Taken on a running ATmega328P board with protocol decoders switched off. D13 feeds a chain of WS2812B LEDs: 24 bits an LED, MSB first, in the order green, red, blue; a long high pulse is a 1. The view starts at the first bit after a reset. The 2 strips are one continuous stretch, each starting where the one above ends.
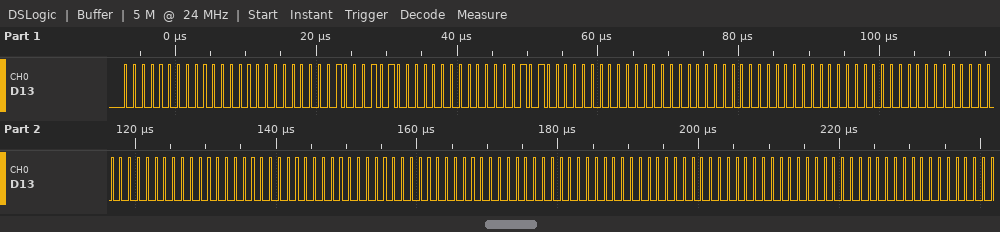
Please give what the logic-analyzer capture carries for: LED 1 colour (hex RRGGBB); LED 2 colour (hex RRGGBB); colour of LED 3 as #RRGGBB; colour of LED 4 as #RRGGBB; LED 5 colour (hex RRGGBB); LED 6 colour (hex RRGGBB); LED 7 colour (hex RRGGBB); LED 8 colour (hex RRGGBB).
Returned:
#000000
#008A05
#000000
#000000
#000000
#000000
#000000
#000000
